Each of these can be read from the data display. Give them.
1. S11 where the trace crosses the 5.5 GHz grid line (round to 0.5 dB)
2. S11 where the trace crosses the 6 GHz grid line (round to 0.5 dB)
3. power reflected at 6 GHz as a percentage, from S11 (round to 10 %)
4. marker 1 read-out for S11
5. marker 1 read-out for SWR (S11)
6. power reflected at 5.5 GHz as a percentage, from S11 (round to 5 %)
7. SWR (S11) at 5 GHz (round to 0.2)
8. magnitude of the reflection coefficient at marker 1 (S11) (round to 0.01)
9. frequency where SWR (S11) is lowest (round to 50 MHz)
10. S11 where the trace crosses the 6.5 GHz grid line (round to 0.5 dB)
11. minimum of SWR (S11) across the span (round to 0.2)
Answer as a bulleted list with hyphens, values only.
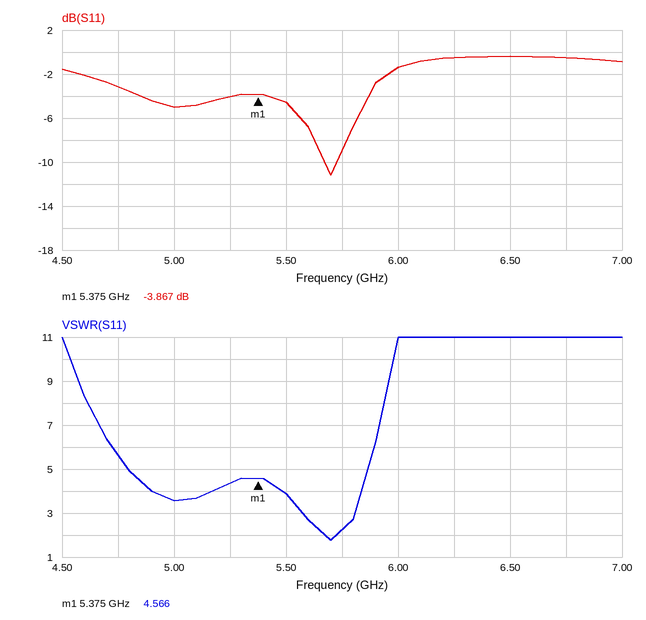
- -4.5 dB
- -1.5 dB
- 70 %
- -3.867 dB
- 4.566
- 35 %
- 3.6
- 0.64
- 5.70 GHz
- -0.5 dB
- 1.8
